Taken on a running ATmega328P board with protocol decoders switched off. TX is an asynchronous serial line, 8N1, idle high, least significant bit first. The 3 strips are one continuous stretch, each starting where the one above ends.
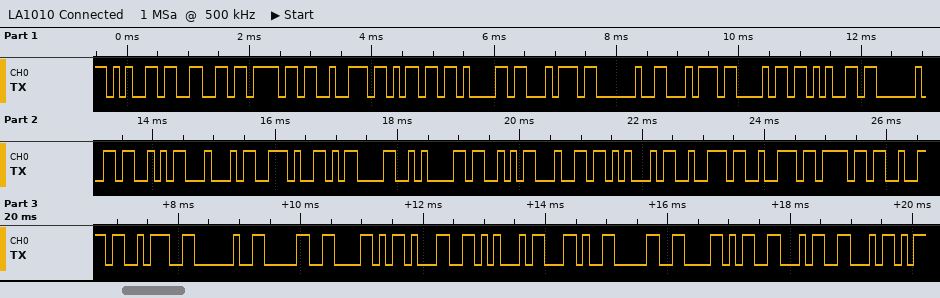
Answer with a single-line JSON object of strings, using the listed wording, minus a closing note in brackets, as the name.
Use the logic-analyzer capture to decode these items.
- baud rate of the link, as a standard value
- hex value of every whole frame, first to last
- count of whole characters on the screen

{"baud rate of the link, as a standard value": "9600 baud", "hex value of every whole frame, first to last": "65 66 6F 72 6D 61 74 20 74 68 65 20 53 44 2E 0D 0A 53 64 45 72 72 6F 72 3A 20 30 58 31 45 2C 30 58 46 46", "count of whole characters on the screen": "35"}
